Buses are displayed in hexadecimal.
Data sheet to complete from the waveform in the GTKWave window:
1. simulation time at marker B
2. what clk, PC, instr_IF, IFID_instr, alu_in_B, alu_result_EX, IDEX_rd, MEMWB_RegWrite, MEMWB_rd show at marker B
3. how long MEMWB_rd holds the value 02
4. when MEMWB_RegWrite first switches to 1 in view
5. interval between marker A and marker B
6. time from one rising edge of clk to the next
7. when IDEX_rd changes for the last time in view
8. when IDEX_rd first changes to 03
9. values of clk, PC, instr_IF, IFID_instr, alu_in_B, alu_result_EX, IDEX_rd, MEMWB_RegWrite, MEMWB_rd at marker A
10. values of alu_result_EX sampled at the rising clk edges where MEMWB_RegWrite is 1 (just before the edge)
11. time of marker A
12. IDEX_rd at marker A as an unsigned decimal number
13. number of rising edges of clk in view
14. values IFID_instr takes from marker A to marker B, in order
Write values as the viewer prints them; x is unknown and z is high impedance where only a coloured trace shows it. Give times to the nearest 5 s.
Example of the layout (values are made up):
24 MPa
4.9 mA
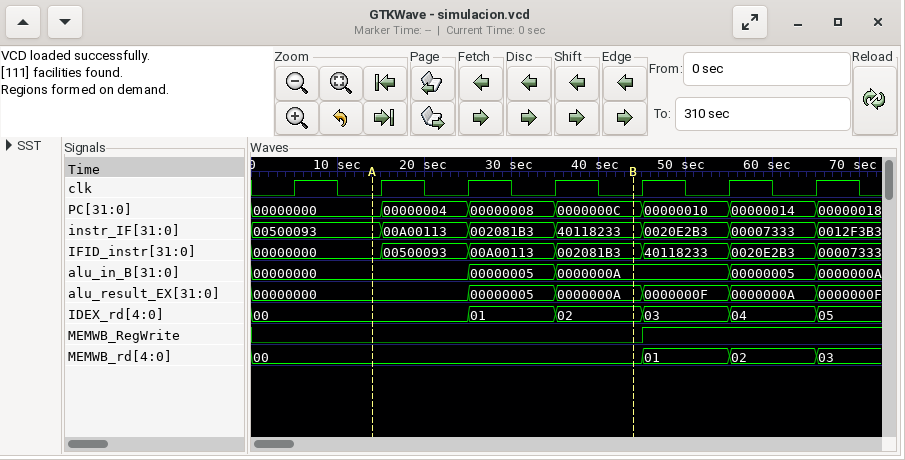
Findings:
45 s
clk=0, PC=0000000C, instr_IF=40118233, IFID_instr=002081B3, alu_in_B=0000000A, alu_result_EX=0000000A, IDEX_rd=02, MEMWB_RegWrite=0, MEMWB_rd=00
10 s
45 s
30 s
10 s
65 s
45 s
clk=0, PC=00000000, instr_IF=00500093, IFID_instr=00000000, alu_in_B=00000000, alu_result_EX=00000000, IDEX_rd=00, MEMWB_RegWrite=0, MEMWB_rd=00
0000000F, 0000000A
15 s
0
7
00000000, 00500093, 00A00113, 002081B3
